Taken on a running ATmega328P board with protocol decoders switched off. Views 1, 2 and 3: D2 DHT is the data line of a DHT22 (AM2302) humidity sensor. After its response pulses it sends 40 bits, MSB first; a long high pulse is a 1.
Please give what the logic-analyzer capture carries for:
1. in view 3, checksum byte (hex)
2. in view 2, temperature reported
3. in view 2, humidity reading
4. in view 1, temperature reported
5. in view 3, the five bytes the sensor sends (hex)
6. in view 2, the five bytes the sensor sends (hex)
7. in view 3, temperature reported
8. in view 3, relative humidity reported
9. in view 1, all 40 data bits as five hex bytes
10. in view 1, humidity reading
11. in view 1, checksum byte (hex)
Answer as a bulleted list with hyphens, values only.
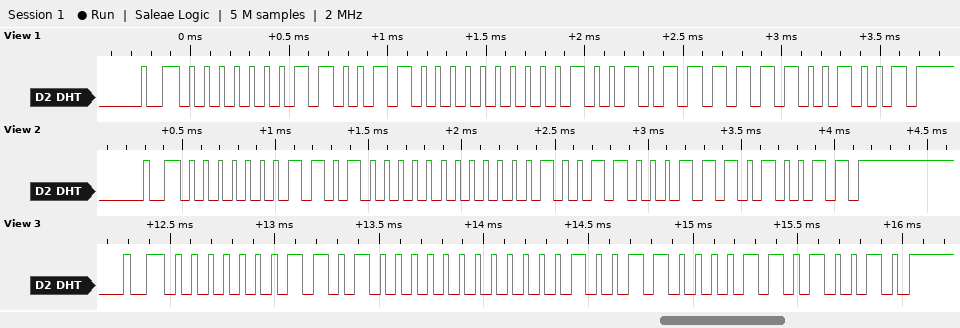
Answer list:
- 0xD2
- 30.5 °C
- 41.6 %
- 30.3 °C
- 01 A0 01 30 D2
- 01 A0 01 31 D3
- 30.4 °C
- 41.6 %
- 01 98 01 2F C9
- 40.8 %
- 0xC9
